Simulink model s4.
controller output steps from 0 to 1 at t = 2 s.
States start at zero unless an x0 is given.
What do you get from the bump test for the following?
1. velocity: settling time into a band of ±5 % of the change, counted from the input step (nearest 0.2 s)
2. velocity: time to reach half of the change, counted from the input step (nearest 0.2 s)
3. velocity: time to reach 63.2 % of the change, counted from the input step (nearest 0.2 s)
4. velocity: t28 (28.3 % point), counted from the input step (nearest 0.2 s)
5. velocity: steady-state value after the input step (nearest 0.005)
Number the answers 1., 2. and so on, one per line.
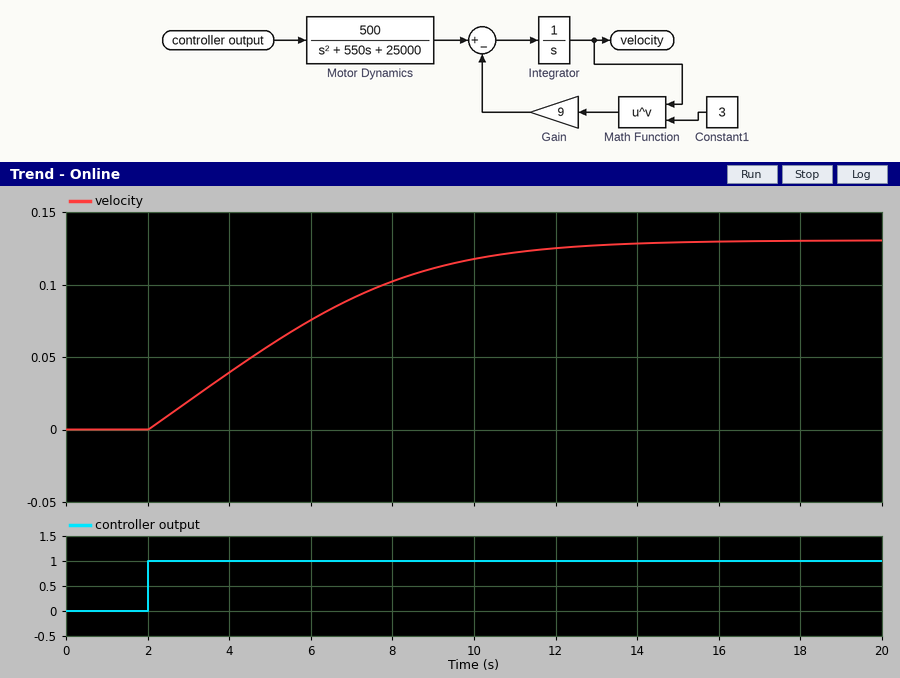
1. 9.6 s
2. 3.4 s
3. 4.4 s
4. 1.8 s
5. 0.130
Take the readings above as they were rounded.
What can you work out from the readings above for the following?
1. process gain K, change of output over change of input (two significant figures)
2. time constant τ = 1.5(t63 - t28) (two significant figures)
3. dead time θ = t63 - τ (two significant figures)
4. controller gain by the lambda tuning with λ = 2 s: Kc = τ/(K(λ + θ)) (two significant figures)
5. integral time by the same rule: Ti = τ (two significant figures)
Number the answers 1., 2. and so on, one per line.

1. 0.13
2. 3.9 s
3. 0.50 s
4. 12
5. 3.9 s
